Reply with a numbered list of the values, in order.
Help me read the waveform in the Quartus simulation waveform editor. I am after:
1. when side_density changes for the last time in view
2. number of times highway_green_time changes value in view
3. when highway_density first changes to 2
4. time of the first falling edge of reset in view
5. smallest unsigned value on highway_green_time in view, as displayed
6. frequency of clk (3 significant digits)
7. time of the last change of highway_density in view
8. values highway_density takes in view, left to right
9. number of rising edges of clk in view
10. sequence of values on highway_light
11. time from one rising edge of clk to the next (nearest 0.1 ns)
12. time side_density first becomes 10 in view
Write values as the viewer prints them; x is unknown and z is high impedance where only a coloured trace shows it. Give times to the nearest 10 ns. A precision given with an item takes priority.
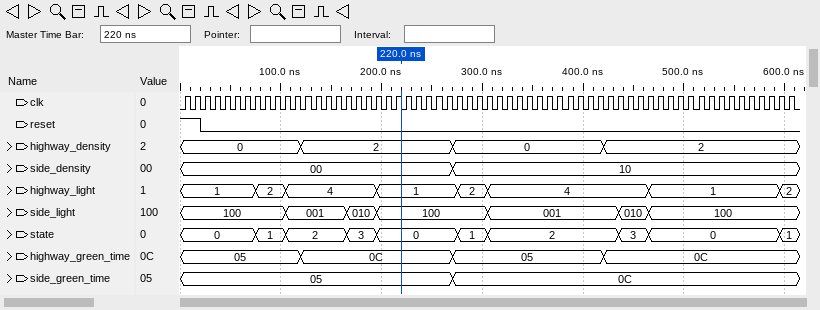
1. 270 ns
2. 3
3. 120 ns
4. 20 ns
5. 05
6. 100 MHz
7. 420 ns
8. 0, 2, 0, 2
9. 61
10. 1, 2, 4, 1, 2, 4, 1, 2
11. 10 ns
12. 270 ns
